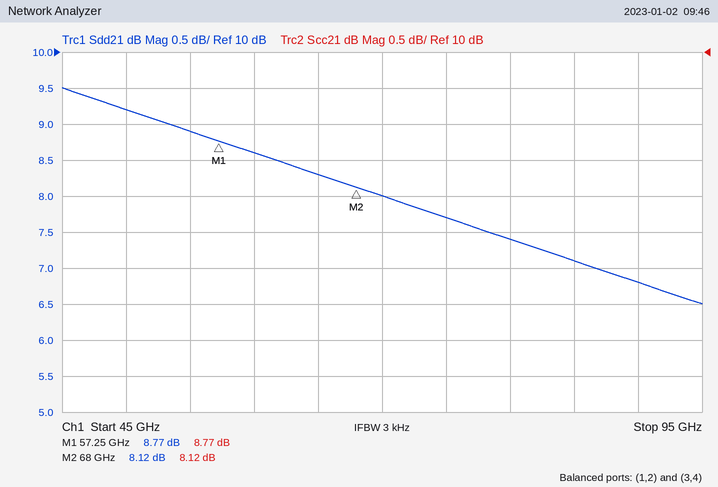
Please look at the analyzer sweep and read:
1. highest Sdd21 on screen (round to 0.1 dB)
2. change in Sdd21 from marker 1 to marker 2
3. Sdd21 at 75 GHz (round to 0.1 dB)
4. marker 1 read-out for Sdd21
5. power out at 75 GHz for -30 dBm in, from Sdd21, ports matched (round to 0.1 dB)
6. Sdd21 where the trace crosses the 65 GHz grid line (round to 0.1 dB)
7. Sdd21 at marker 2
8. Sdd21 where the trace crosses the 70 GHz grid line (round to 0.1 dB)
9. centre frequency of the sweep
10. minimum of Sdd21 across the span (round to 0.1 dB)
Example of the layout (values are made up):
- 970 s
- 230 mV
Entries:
- 9.5 dB
- -0.65 dB
- 7.7 dB
- 8.77 dB
- -22.3 dBm
- 8.3 dB
- 8.12 dB
- 8.0 dB
- 70 GHz
- 6.5 dB
